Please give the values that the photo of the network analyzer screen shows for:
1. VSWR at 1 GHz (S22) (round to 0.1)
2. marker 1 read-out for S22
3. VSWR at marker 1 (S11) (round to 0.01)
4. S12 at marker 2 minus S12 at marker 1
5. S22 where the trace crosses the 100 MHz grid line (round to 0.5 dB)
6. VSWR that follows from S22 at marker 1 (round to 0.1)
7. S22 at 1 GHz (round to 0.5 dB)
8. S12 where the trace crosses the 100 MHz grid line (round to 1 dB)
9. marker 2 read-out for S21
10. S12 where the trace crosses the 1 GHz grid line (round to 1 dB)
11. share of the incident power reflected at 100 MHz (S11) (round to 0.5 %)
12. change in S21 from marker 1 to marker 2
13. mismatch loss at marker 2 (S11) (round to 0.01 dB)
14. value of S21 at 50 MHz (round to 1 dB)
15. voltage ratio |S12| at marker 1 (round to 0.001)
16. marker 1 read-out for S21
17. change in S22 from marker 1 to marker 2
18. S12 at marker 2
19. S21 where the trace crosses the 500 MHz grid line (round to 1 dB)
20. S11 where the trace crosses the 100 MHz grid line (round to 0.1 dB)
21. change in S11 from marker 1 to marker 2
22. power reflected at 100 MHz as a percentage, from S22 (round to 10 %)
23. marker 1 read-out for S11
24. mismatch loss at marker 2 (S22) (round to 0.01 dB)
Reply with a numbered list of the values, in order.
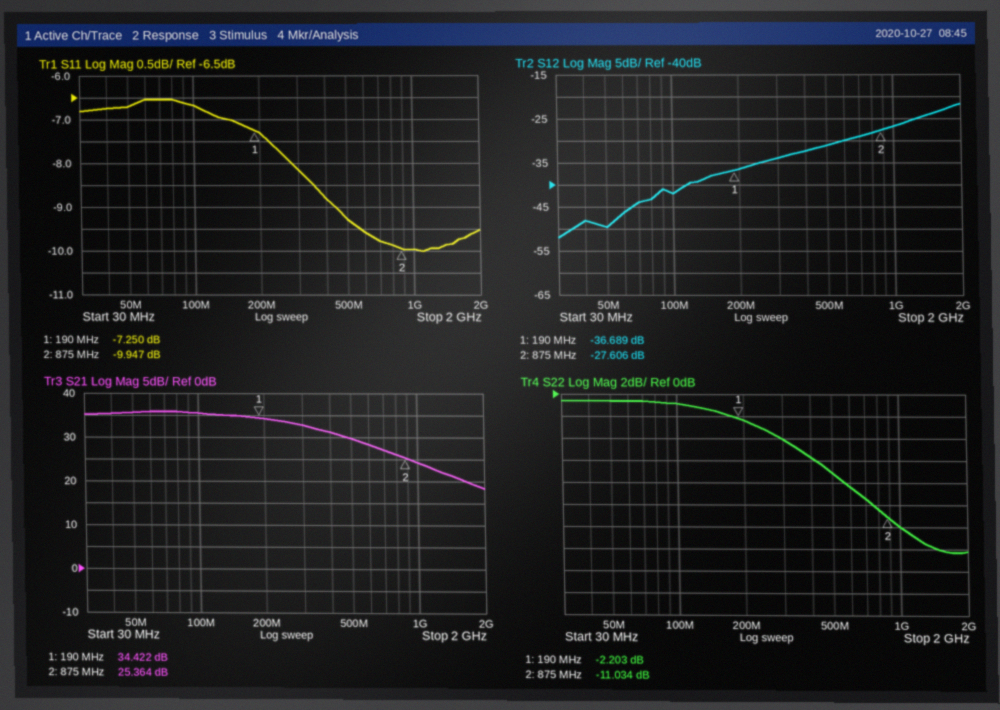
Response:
1. 1.7
2. -2.203 dB
3. 2.53
4. 9.083 dB
5. -1.0 dB
6. 7.9
7. -12.0 dB
8. -42 dB
9. 25.364 dB
10. -27 dB
11. 21.5 %
12. -9.058 dB
13. 0.46 dB
14. 36 dB
15. 0.015
16. 34.422 dB
17. -8.831 dB
18. -27.606 dB
19. 30 dB
20. -6.7 dB
21. -2.697 dB
22. 80 %
23. -7.250 dB
24. 0.36 dB
